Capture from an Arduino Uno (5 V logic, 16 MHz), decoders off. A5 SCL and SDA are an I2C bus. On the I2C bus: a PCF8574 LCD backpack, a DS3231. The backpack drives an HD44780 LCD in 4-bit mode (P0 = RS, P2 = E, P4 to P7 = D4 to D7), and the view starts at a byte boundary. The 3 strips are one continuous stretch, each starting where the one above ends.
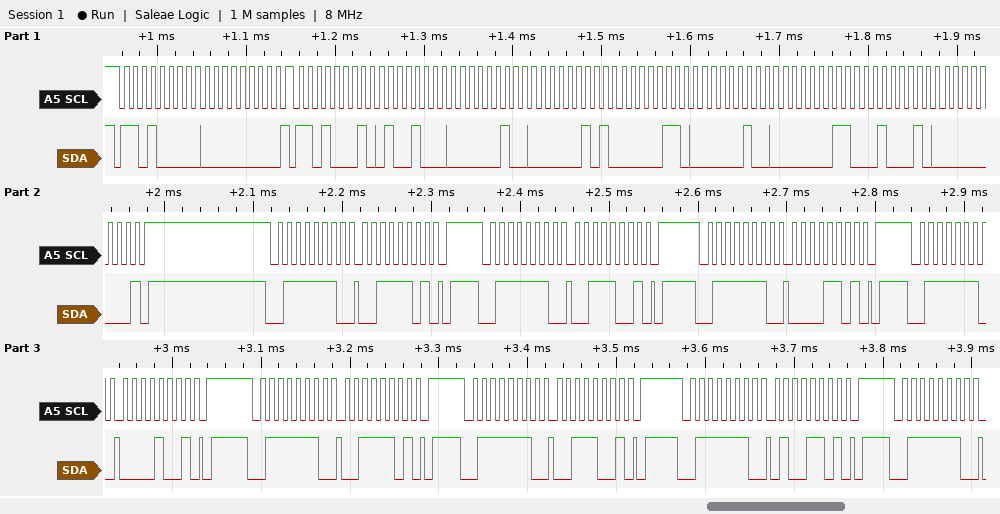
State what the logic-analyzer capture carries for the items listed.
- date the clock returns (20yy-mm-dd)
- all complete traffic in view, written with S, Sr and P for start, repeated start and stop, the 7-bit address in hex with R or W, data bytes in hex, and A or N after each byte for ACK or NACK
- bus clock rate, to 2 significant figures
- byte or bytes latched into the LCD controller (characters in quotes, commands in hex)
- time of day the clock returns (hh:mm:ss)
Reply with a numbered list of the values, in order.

1. 2022-03-04
2. S 68W A 00 A Sr 68R A 48 A 04 A 05 A 06 A 04 A 03 A 22 A 00 N P S 3FW A 3D A P S 3FW A 39 A P S 3FW A 0D A P S 3FW A 09 A P S 3FW A 3D A P S 3FW A 39 A P S 3FW A 4D A P S 3FW A
3. 100 kHz
4. '0'
5. 05:04:48
